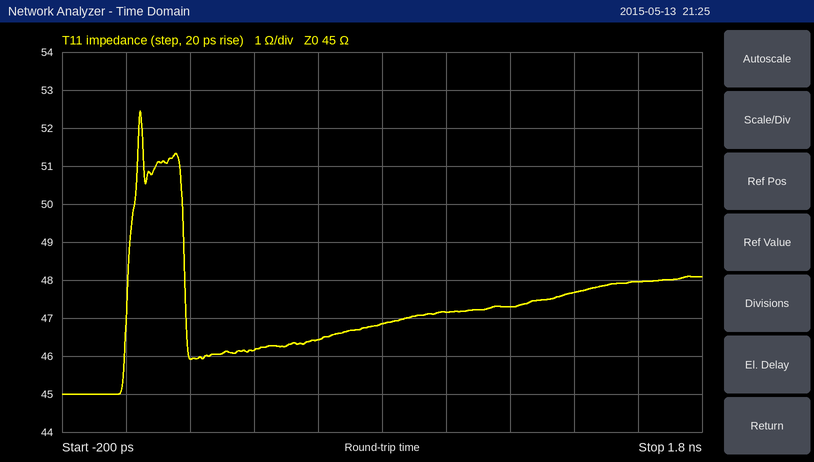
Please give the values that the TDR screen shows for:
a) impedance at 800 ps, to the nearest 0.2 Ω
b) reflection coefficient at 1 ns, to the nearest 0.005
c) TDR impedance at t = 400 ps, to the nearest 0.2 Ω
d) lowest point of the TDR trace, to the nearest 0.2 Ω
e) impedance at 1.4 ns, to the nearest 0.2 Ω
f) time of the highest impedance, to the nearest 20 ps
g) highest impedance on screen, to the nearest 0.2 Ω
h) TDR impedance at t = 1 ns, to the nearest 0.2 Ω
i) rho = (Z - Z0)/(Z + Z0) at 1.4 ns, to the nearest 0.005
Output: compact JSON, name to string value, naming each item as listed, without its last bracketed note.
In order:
{"impedance at 800 ps, to the nearest 0.2 Ω": "46.8 Ω", "reflection coefficient at 1 ns, to the nearest 0.005": "+0.025", "TDR impedance at t = 400 ps, to the nearest 0.2 Ω": "46.2 Ω", "lowest point of the TDR trace, to the nearest 0.2 Ω": "45.0 Ω", "impedance at 1.4 ns, to the nearest 0.2 Ω": "47.6 Ω", "time of the highest impedance, to the nearest 20 ps": "40 ps", "highest impedance on screen, to the nearest 0.2 Ω": "52.4 Ω", "TDR impedance at t = 1 ns, to the nearest 0.2 Ω": "47.2 Ω", "rho = (Z - Z0)/(Z + Z0) at 1.4 ns, to the nearest 0.005": "+0.030"}
